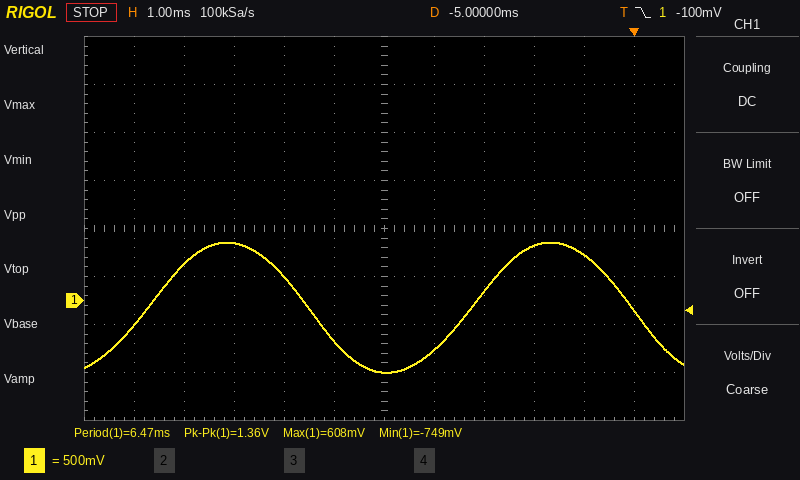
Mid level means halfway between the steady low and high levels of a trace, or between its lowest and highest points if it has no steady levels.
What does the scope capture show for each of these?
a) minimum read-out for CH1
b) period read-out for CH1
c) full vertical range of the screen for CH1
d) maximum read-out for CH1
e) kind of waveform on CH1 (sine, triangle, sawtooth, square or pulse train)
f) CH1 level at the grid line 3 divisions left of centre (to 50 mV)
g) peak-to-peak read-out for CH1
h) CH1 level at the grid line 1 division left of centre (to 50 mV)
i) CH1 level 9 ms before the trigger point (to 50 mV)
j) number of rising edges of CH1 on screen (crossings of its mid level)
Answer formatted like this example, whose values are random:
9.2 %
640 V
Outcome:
-749 mV
6.47 ms
4 V
608 mV
sine
600 mV
1.36 V
-400 mV
400 mV
2
